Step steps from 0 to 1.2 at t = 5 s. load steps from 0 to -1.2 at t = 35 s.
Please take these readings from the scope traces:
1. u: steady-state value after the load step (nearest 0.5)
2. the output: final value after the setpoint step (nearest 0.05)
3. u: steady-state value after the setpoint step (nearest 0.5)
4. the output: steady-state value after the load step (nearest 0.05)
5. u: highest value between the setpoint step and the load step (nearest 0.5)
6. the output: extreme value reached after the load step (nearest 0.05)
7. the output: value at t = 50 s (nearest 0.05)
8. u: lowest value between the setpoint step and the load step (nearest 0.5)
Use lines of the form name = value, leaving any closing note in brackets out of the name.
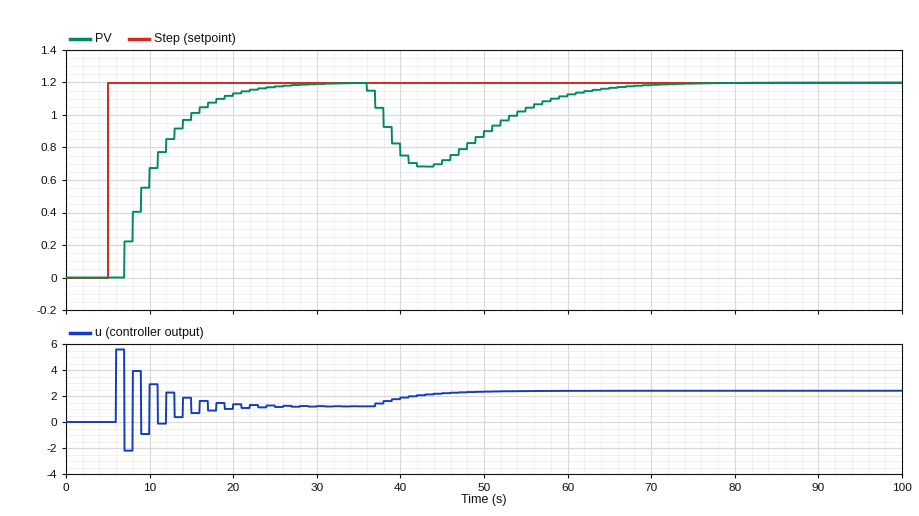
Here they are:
u: steady-state value after the load step = 2.5
the output: final value after the setpoint step = 1.20
u: steady-state value after the setpoint step = 1.0
the output: steady-state value after the load step = 1.20
u: highest value between the setpoint step and the load step = 5.5
the output: extreme value reached after the load step = 0.70
the output: value at t = 50 s = 0.90
u: lowest value between the setpoint step and the load step = -2.0
